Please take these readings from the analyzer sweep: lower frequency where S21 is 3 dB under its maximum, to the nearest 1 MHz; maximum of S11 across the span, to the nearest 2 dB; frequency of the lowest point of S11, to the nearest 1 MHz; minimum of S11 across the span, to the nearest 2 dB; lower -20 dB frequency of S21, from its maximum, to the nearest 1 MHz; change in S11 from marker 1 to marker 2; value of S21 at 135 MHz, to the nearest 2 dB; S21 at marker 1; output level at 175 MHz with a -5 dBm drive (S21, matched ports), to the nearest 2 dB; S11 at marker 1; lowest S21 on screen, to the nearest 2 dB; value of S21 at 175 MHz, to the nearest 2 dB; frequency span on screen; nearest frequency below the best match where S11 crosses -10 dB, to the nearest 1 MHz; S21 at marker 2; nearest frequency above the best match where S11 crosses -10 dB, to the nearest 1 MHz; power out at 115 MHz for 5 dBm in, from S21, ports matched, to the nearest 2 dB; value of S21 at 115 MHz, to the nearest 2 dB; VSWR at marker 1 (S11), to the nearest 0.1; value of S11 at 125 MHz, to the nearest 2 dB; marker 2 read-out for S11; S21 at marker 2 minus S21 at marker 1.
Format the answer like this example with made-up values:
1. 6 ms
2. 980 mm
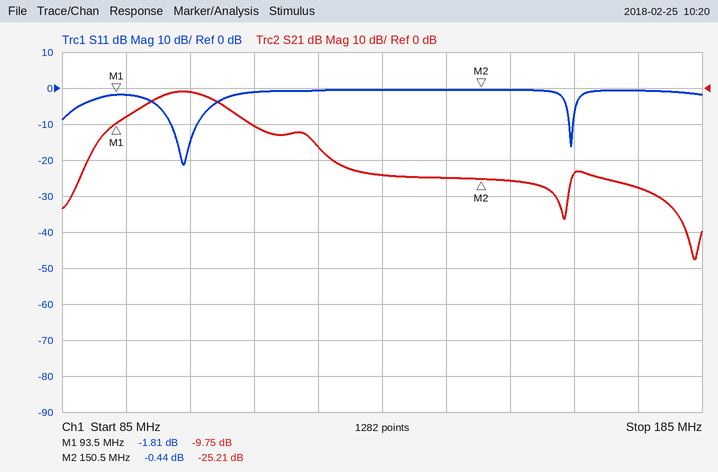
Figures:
1. 99 MHz
2. 0 dB
3. 104 MHz
4. -22 dB
5. 89 MHz
6. 1.37 dB
7. -24 dB
8. -9.75 dB
9. -32 dBm
10. -1.81 dB
11. -48 dB
12. -28 dB
13. 100 MHz
14. 102 MHz
15. -25.21 dB
16. 106 MHz
17. -6 dBm
18. -10 dB
19. 9.6
20. 0 dB
21. -0.44 dB
22. -15.46 dB
